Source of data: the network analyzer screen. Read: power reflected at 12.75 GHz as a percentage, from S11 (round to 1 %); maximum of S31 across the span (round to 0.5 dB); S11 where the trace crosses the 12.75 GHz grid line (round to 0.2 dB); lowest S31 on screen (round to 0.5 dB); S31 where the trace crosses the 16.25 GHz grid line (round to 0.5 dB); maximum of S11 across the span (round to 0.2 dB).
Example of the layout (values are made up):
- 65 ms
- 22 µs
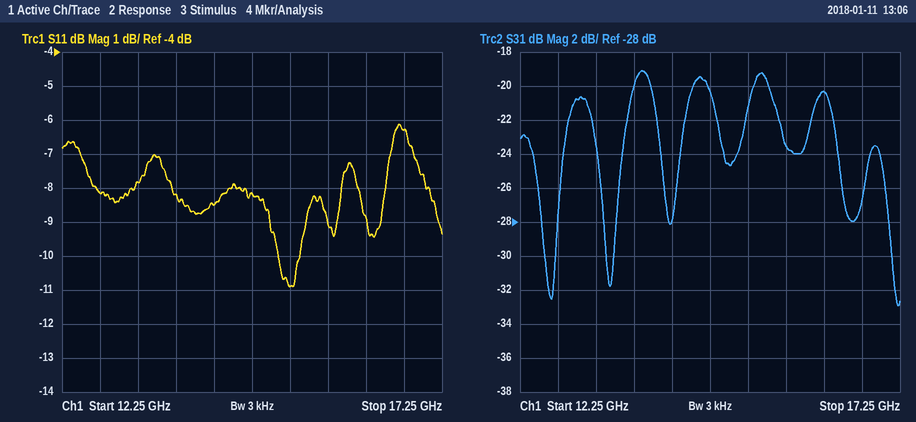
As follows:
- 15 %
- -19.0 dB
- -8.2 dB
- -33.0 dB
- -20.5 dB
- -6.2 dB
